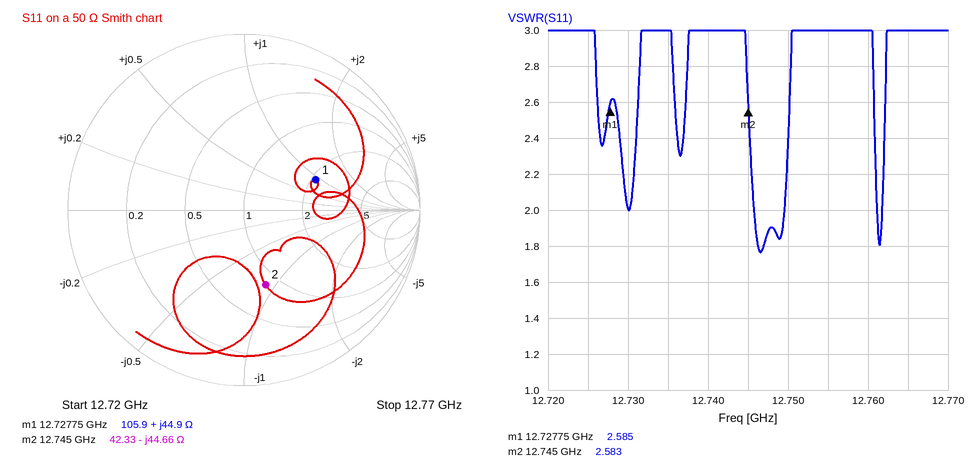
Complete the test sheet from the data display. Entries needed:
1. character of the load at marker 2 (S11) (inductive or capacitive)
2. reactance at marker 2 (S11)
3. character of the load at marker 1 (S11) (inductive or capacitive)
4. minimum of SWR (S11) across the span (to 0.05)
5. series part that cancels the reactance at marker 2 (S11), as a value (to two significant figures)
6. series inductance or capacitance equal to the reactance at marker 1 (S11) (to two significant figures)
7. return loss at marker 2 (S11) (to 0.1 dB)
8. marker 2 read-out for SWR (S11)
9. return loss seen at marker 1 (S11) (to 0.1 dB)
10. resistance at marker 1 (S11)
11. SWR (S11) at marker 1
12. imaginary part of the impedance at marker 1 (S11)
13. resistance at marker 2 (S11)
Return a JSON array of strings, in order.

["capacitive", "-44.66 Ω", "inductive", "1.75", "560 pH", "560 pH", "7.1 dB", "2.583", "7.1 dB", "105.9 Ω", "2.585", "+44.9 Ω", "42.33 Ω"]
